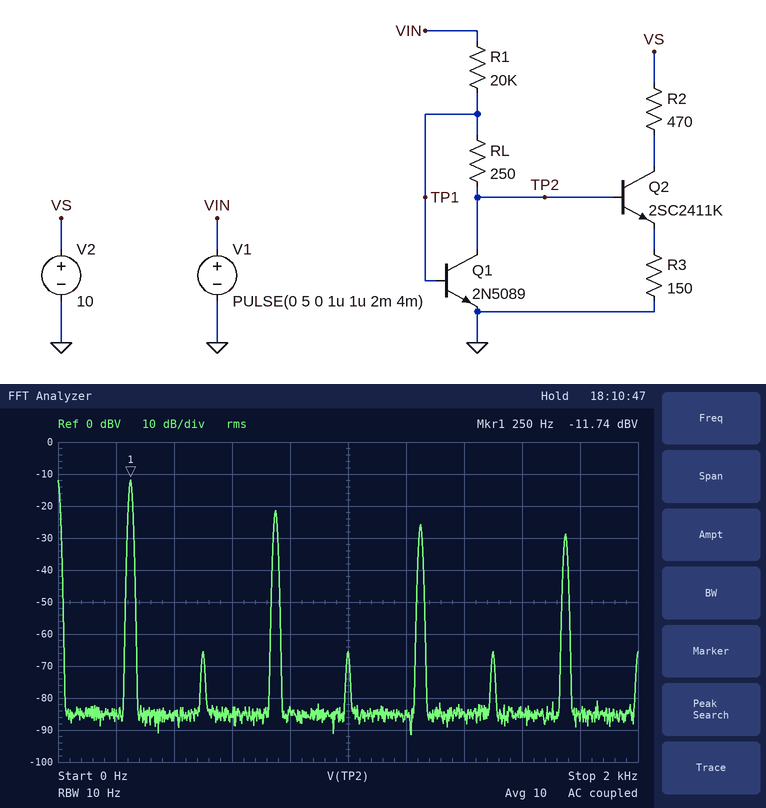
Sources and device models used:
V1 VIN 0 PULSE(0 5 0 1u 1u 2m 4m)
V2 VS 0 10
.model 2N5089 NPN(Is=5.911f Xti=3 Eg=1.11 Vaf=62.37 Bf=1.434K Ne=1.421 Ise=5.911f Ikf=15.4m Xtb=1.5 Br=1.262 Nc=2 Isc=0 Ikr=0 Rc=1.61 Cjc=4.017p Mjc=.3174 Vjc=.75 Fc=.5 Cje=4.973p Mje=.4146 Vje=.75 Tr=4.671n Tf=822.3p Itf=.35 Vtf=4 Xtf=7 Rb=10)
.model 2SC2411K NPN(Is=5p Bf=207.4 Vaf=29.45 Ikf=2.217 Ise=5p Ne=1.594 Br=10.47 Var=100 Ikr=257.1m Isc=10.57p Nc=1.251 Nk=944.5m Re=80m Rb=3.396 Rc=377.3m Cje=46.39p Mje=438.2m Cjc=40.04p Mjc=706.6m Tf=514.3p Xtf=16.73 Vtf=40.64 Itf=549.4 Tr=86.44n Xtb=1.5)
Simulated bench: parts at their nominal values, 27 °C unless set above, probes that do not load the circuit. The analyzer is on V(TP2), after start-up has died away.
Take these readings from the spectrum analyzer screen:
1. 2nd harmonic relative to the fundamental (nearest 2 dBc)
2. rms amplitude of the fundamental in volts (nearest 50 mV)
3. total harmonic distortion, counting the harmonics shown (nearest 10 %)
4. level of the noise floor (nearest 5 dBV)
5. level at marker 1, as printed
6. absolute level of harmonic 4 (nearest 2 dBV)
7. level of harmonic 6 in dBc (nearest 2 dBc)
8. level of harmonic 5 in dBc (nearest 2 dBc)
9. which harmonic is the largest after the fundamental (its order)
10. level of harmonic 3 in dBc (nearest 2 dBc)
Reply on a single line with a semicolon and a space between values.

-54 dBc; 250 mV; 40 %; -85 dBV; -11.74 dBV; -66 dBV; -54 dBc; -14 dBc; 3; -10 dBc
